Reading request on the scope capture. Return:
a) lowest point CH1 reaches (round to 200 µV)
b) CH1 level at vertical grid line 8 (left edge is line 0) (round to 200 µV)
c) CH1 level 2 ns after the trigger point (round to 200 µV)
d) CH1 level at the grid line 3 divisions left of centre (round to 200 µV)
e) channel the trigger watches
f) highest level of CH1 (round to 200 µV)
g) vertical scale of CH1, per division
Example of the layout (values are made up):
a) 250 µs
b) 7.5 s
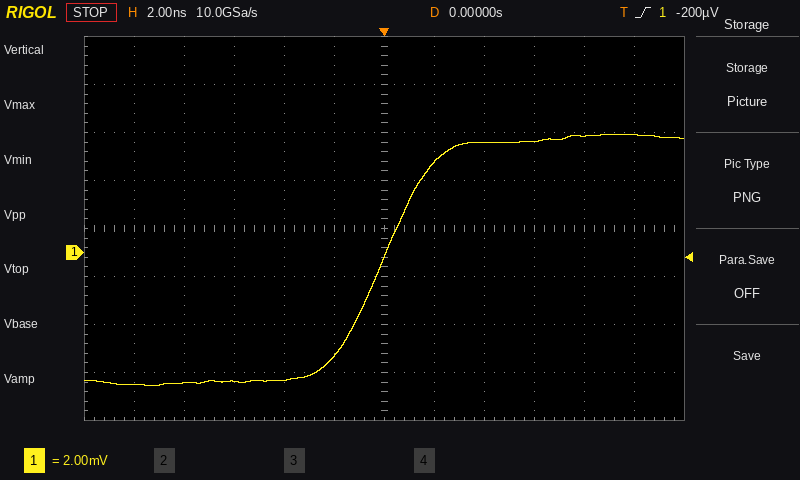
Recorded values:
a) -5.6 mV
b) 4.6 mV
c) 3.8 mV
d) -5.4 mV
e) CH1
f) 5.0 mV
g) 2 mV
